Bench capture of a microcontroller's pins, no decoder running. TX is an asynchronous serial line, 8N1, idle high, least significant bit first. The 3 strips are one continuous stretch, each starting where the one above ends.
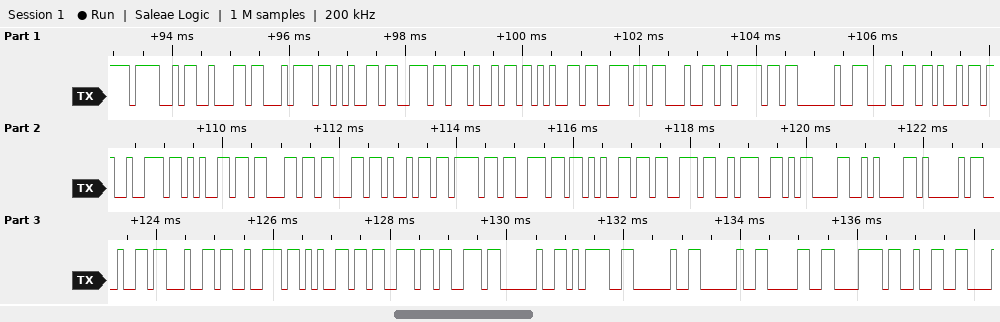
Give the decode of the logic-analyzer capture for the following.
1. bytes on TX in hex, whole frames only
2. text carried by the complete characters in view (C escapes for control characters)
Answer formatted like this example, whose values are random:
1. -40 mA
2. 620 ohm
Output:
1. 4F 62 74 65 6E 69 65 6E 64 6F 20 64 69 72 65 63 63 69 6F 6E 65 73 3A 0D 0A 41 64 64 72 65 73 73 20 3D 20 20 30 78 32
2. "Obteniendo direcciones:\r\nAddress =  0x2"
